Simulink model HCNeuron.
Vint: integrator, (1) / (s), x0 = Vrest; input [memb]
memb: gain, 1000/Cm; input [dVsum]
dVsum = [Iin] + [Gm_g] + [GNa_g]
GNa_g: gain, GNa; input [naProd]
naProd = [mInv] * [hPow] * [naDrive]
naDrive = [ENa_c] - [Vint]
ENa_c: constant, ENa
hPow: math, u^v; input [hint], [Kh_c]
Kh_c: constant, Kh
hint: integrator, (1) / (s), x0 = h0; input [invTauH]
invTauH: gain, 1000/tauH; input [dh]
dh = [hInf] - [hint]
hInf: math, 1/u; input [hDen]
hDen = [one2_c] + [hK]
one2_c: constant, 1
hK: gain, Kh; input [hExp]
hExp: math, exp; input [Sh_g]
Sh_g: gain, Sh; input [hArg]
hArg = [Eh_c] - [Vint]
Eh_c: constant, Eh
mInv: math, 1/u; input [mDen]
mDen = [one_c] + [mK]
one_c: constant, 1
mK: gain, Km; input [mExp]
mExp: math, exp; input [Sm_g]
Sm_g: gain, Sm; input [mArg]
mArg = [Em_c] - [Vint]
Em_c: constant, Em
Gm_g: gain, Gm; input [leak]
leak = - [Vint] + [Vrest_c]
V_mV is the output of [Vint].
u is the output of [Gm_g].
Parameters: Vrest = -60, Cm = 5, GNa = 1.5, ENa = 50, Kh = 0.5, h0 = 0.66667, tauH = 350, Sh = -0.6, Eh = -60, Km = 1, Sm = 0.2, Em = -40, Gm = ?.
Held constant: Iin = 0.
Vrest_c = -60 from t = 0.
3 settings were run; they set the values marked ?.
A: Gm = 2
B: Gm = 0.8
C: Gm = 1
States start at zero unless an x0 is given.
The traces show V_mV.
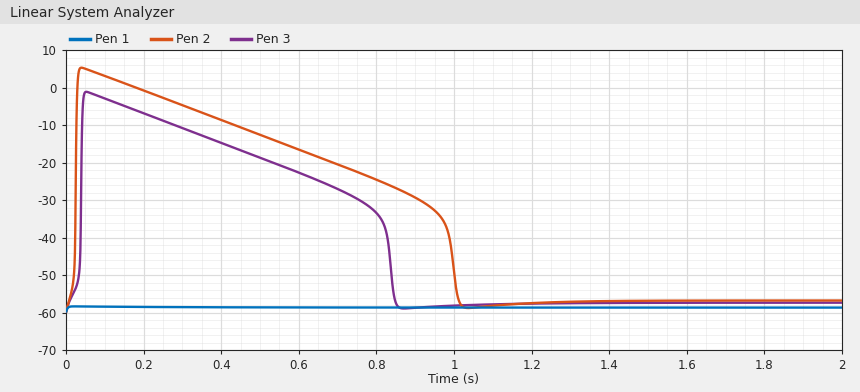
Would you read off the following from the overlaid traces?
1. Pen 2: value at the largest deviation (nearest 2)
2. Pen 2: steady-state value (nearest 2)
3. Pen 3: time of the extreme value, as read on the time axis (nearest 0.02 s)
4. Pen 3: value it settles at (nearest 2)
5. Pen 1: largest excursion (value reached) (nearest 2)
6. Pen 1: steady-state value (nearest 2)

6
-56
0.06 s
-58
-58
-58
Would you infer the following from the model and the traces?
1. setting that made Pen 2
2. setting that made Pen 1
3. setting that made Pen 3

B
A
C
